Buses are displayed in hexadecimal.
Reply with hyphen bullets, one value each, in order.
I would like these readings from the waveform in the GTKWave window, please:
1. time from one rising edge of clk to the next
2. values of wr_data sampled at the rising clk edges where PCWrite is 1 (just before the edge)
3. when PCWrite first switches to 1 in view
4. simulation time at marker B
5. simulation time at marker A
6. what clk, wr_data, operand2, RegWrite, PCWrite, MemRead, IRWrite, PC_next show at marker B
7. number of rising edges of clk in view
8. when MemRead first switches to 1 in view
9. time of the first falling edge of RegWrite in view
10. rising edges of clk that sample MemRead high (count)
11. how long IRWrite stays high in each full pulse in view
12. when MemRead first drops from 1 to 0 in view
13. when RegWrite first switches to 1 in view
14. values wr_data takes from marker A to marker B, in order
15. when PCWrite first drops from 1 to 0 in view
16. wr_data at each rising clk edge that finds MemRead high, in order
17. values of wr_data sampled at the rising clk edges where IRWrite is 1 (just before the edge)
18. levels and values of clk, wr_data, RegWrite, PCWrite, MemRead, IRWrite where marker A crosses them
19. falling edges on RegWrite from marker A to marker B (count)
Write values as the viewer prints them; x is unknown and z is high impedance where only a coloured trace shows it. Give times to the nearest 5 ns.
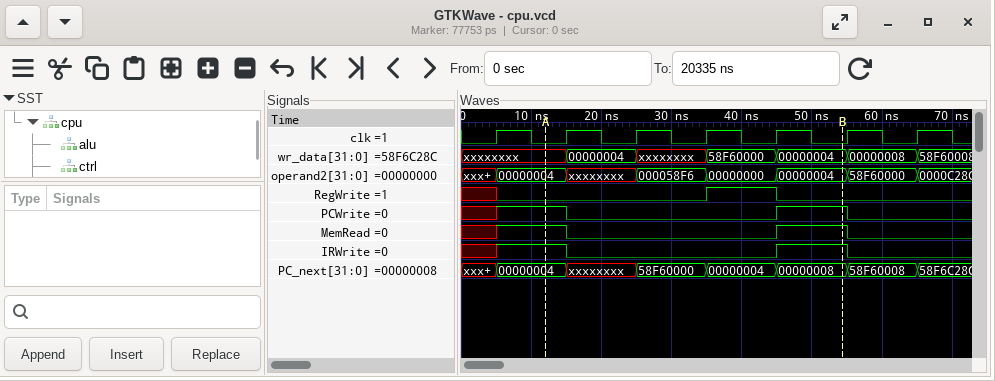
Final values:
- 10 ns
- xxxxxxxx, 00000004
- 5 ns
- 55 ns
- 10 ns
- clk=0, wr_data=00000004, operand2=00000004, RegWrite=0, PCWrite=1, MemRead=1, IRWrite=1, PC_next=00000008
- 7
- 5 ns
- 45 ns
- 2
- 10 ns
- 15 ns
- 35 ns
- xxxxxxxx, 00000004, xxxxxxxx, 58F60000, 00000004
- 15 ns
- xxxxxxxx, 00000004
- xxxxxxxx, 00000004
- clk=0, wr_data=xxxxxxxx, RegWrite=0, PCWrite=1, MemRead=1, IRWrite=1
- 1
